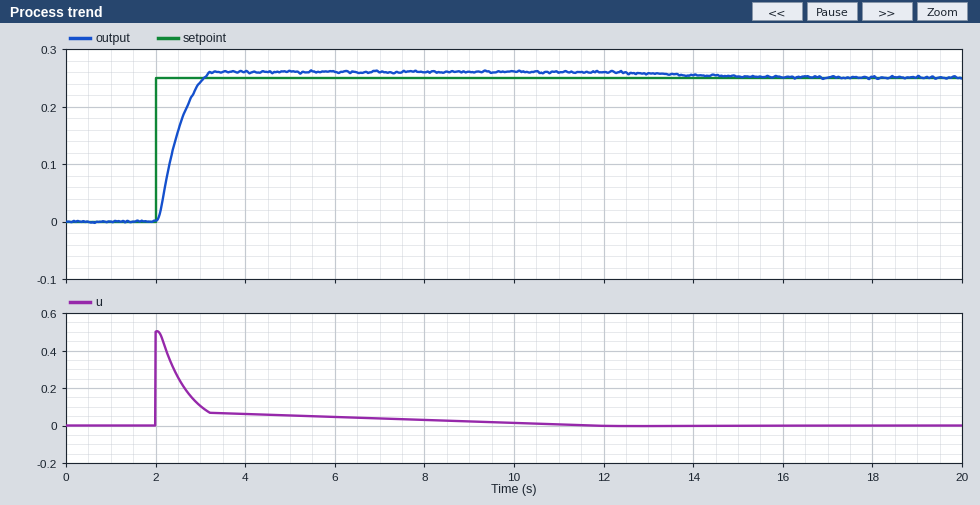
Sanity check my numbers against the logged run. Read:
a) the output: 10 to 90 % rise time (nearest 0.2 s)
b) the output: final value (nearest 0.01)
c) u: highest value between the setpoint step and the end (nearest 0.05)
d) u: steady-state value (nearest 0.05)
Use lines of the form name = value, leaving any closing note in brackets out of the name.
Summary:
the output: 10 to 90 % rise time = 0.8 s
the output: final value = 0.25
u: highest value between the setpoint step and the end = 0.50
u: steady-state value = 0.00
